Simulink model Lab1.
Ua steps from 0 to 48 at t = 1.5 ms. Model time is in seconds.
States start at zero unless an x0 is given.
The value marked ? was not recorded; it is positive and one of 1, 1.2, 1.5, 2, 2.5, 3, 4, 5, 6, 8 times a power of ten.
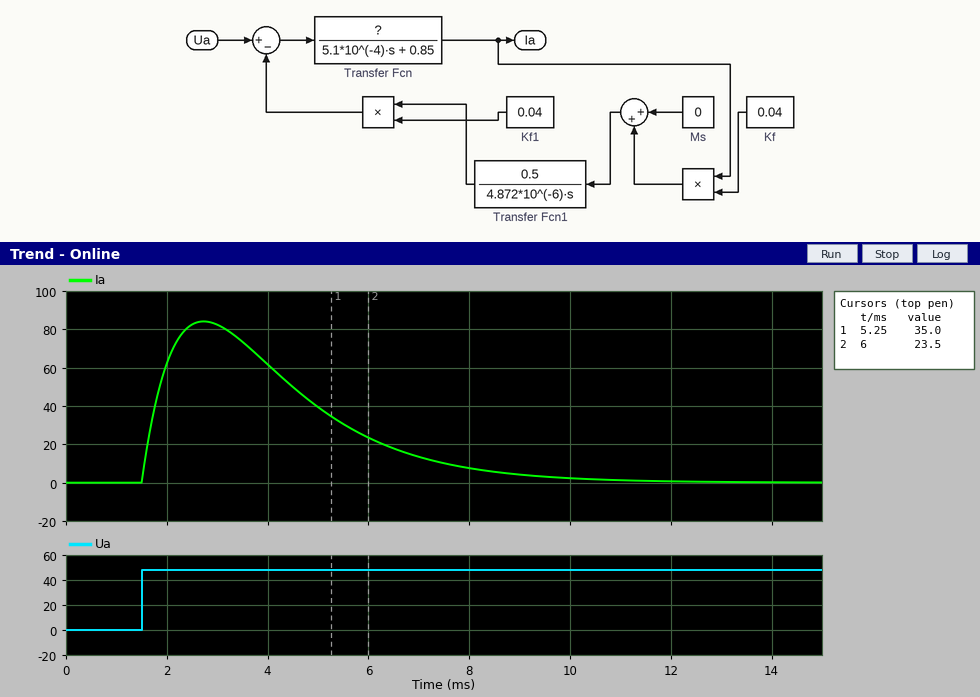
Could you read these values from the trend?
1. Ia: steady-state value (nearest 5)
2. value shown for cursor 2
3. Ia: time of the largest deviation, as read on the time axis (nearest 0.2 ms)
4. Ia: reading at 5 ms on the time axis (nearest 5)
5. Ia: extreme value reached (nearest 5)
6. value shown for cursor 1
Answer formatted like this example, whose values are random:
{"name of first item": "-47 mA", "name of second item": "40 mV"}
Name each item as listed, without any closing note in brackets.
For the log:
{"Ia: steady-state value": "0", "value shown for cursor 2": "23.5", "Ia: time of the largest deviation, as read on the time axis": "2.8 ms", "Ia: reading at 5 ms on the time axis": "40", "Ia: extreme value reached": "85", "value shown for cursor 1": "35.0"}
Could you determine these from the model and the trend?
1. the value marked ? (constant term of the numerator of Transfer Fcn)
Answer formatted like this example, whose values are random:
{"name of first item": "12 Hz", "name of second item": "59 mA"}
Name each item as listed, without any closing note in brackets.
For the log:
{"the value marked ?": "2"}
